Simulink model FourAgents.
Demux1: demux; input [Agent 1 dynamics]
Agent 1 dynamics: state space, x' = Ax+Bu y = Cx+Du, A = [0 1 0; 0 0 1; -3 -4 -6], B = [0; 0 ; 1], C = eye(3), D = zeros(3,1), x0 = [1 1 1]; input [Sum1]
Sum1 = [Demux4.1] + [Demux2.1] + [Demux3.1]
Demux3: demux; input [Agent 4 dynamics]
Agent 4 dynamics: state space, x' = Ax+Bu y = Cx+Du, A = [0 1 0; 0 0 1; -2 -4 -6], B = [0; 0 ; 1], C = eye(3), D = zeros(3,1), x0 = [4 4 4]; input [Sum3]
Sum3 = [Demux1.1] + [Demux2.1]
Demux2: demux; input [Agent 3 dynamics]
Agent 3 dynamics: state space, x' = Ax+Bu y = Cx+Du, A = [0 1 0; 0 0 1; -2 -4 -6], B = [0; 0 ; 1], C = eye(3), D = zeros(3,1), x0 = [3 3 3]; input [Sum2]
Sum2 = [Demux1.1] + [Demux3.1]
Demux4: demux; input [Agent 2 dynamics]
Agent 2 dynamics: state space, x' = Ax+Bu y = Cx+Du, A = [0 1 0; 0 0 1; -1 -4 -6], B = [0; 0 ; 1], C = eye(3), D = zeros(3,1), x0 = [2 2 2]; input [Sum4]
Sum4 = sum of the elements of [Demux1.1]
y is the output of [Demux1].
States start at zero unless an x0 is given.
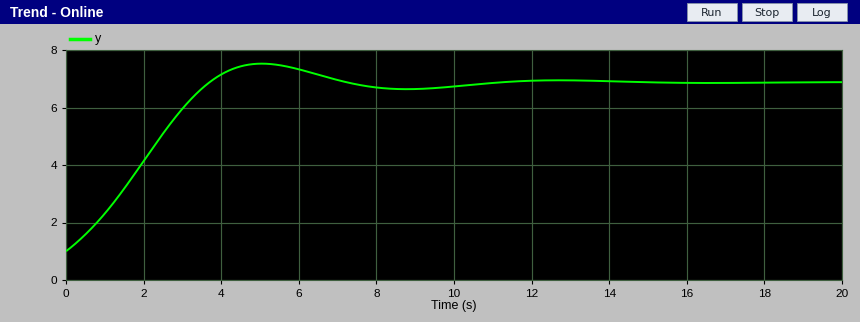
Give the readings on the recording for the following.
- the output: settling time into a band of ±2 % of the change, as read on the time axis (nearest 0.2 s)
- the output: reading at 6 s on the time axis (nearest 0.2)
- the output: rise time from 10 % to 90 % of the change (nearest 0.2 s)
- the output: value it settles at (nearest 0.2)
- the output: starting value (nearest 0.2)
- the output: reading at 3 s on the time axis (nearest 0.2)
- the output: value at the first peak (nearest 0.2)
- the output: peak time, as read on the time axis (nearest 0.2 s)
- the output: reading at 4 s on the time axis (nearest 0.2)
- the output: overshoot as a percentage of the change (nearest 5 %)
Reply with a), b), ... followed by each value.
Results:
a) 10.2 s
b) 7.4
c) 2.8 s
d) 6.8
e) 1.0
f) 6.0
g) 7.6
h) 5.0 s
i) 7.2
j) 10 %
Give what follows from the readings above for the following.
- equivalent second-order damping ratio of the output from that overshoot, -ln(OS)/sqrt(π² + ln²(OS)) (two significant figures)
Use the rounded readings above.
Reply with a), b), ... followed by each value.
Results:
a) 0.59
